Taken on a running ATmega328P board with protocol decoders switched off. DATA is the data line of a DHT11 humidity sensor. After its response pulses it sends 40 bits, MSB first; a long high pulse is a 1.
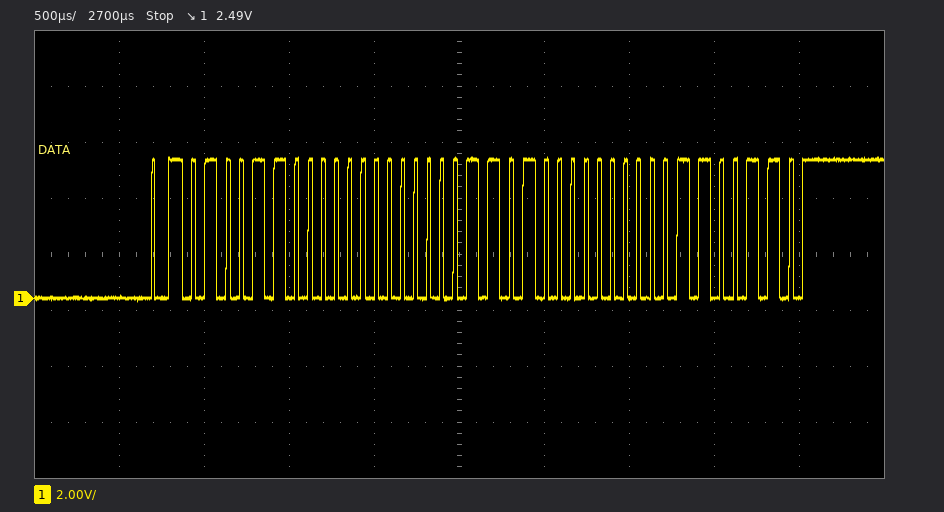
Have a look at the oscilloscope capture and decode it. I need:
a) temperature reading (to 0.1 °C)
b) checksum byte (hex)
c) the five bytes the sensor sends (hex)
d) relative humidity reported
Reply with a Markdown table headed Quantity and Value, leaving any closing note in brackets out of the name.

| Quantity | Value |
|---|---|
| temperature reading | 26.0 °C |
| checksum byte | 0x66 |
| the five bytes the sensor sends | 4C 00 1A 00 66 |
| relative humidity reported | 76 % |
